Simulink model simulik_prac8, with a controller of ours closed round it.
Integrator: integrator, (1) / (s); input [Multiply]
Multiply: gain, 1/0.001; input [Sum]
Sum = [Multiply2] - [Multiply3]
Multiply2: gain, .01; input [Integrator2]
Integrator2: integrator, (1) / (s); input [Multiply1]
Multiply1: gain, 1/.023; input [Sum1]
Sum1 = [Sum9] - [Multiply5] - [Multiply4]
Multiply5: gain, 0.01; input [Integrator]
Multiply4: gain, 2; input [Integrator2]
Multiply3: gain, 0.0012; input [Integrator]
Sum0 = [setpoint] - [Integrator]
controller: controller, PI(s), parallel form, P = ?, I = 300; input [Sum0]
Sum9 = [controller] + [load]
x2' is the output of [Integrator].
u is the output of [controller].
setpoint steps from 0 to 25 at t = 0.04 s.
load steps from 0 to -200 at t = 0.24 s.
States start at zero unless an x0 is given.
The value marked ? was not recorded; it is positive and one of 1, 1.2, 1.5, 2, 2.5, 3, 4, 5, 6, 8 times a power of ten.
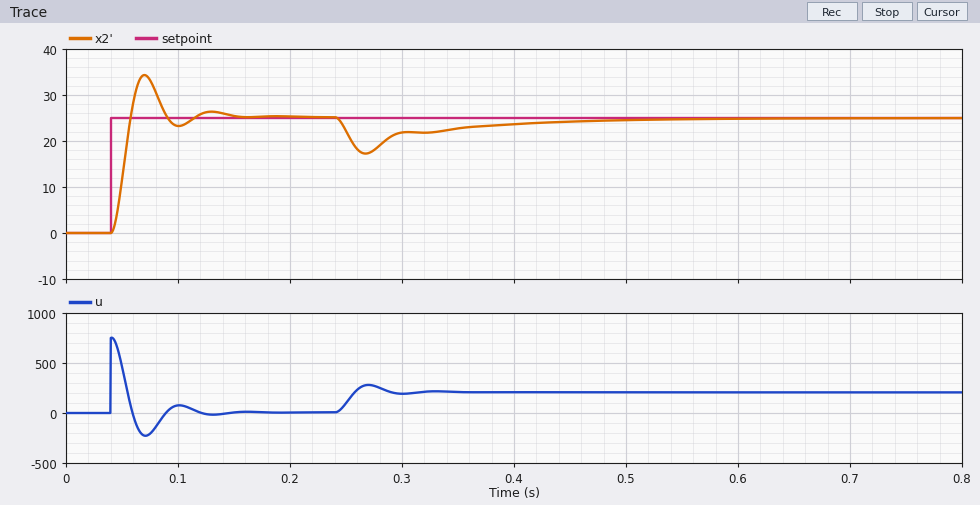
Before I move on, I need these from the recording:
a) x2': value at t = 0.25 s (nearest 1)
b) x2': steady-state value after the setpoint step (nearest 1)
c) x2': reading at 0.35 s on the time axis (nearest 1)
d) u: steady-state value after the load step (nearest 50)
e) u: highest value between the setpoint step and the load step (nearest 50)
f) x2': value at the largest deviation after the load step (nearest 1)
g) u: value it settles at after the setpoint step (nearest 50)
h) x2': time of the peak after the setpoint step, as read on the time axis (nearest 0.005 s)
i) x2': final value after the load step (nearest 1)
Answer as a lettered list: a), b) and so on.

a) 22
b) 25
c) 23
d) 200
e) 750
f) 17
g) 0
h) 0.070 s
i) 25
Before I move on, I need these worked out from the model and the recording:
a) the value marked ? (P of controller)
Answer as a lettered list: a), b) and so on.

a) 30
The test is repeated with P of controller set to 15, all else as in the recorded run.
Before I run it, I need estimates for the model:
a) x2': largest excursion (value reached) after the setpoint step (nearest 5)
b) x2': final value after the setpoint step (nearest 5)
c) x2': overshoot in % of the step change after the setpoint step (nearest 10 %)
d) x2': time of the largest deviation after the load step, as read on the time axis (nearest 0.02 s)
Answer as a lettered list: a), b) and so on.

a) 35
b) 25
c) 40 %
d) 0.28 s
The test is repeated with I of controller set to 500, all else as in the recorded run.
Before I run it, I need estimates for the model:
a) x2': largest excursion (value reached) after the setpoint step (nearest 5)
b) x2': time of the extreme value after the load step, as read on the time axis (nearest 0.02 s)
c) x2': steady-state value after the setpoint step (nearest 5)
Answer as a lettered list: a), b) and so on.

a) 35
b) 0.26 s
c) 25
